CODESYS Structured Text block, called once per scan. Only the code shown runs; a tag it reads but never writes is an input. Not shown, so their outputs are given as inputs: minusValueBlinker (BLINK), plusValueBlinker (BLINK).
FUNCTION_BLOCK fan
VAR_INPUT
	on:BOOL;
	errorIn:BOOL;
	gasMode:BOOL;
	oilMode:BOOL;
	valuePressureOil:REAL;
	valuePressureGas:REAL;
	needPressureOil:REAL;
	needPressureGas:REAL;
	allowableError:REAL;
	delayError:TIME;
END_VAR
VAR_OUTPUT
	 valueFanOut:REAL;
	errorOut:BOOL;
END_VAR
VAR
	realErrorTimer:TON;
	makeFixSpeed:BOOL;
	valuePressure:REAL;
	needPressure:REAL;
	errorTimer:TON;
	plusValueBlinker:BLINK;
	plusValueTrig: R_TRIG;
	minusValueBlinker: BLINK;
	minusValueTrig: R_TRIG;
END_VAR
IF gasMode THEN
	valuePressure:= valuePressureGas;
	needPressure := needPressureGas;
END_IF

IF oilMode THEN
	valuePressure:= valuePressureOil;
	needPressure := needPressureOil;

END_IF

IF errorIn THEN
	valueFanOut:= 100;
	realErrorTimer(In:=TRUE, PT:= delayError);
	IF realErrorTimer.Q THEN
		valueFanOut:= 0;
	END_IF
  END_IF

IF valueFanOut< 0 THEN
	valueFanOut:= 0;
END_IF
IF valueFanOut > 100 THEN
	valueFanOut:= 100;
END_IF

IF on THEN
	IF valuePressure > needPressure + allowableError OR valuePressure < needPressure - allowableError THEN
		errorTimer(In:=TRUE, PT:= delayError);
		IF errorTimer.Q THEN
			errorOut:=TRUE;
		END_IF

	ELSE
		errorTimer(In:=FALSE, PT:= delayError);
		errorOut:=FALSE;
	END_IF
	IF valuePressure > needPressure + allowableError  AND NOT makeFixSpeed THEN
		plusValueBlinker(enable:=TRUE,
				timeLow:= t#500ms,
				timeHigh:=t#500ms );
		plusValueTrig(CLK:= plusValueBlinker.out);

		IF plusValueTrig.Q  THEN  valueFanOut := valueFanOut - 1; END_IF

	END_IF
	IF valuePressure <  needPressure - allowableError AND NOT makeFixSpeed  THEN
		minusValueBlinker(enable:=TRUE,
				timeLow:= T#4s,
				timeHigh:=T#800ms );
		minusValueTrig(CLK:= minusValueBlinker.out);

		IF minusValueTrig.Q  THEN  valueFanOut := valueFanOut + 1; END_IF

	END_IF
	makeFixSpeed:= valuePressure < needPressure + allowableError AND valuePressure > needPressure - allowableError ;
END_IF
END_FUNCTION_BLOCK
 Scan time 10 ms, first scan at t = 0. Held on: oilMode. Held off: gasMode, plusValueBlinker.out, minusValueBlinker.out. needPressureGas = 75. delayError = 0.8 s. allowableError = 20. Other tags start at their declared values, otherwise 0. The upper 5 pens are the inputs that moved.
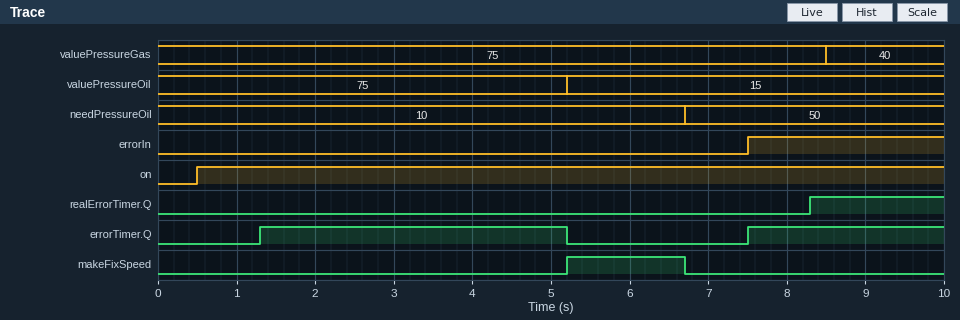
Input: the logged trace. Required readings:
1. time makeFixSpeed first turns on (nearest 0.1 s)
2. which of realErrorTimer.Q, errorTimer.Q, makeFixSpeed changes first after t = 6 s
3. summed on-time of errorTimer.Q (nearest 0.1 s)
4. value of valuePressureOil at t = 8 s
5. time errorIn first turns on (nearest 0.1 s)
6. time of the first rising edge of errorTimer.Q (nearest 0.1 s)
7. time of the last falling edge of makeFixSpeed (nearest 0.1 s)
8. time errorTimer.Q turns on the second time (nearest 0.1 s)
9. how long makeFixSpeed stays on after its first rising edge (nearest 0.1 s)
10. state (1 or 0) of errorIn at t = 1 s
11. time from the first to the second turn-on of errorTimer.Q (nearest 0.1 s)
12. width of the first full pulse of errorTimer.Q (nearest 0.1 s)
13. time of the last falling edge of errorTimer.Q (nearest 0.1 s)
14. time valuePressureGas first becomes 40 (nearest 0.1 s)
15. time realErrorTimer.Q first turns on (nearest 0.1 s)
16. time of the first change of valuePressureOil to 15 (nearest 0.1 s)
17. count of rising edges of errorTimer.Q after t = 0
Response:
5.2 s
makeFixSpeed
6.4 s
15
7.5 s
1.3 s
6.7 s
7.5 s
1.5 s
0
6.2 s
3.9 s
5.2 s
8.5 s
8.3 s
5.2 s
2
